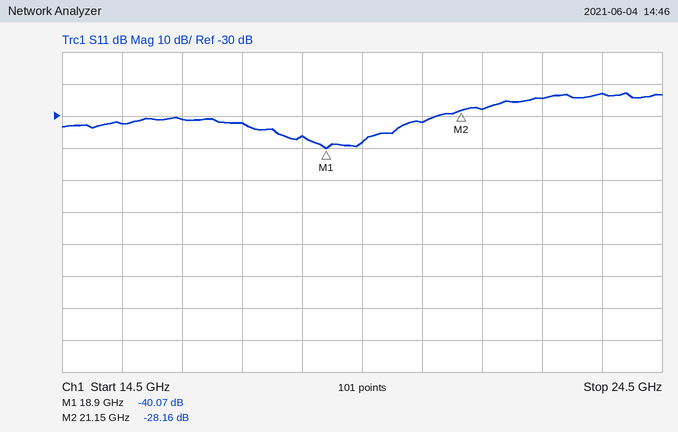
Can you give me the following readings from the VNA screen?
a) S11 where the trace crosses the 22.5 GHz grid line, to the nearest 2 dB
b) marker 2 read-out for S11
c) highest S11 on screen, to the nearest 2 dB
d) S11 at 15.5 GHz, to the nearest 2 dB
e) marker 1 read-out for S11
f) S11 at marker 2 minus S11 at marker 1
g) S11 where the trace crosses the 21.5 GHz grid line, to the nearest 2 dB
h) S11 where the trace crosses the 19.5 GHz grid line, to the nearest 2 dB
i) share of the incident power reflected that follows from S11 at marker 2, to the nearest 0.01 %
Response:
-24 dB
-28.16 dB
-22 dB
-32 dB
-40.07 dB
11.91 dB
-28 dB
-38 dB
0.15 %
